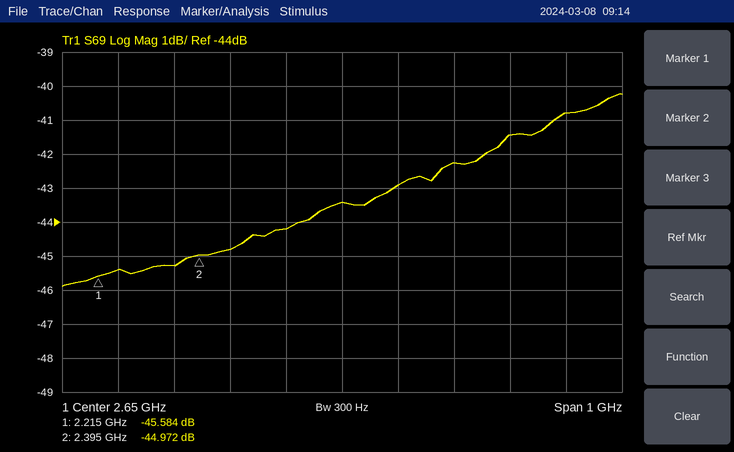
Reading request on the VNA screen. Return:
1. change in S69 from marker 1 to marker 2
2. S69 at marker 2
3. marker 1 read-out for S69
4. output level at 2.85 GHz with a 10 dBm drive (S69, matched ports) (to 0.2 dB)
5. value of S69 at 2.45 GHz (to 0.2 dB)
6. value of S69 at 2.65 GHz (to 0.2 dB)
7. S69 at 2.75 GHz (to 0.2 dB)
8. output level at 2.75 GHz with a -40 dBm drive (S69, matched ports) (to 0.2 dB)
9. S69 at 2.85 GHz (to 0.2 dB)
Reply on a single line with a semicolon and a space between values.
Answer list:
0.612 dB; -44.972 dB; -45.584 dB; -32.2 dBm; -44.8 dB; -43.4 dB; -43.0 dB; -83.0 dBm; -42.2 dB
